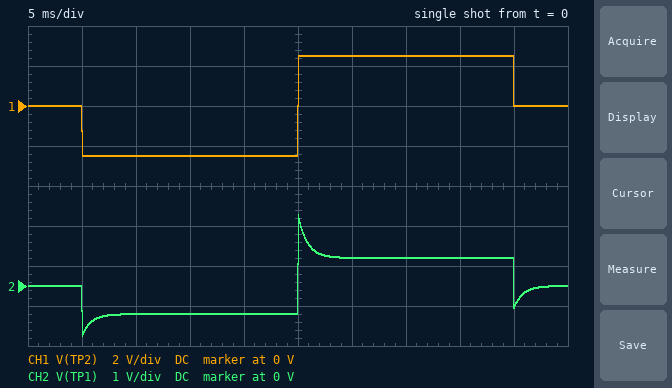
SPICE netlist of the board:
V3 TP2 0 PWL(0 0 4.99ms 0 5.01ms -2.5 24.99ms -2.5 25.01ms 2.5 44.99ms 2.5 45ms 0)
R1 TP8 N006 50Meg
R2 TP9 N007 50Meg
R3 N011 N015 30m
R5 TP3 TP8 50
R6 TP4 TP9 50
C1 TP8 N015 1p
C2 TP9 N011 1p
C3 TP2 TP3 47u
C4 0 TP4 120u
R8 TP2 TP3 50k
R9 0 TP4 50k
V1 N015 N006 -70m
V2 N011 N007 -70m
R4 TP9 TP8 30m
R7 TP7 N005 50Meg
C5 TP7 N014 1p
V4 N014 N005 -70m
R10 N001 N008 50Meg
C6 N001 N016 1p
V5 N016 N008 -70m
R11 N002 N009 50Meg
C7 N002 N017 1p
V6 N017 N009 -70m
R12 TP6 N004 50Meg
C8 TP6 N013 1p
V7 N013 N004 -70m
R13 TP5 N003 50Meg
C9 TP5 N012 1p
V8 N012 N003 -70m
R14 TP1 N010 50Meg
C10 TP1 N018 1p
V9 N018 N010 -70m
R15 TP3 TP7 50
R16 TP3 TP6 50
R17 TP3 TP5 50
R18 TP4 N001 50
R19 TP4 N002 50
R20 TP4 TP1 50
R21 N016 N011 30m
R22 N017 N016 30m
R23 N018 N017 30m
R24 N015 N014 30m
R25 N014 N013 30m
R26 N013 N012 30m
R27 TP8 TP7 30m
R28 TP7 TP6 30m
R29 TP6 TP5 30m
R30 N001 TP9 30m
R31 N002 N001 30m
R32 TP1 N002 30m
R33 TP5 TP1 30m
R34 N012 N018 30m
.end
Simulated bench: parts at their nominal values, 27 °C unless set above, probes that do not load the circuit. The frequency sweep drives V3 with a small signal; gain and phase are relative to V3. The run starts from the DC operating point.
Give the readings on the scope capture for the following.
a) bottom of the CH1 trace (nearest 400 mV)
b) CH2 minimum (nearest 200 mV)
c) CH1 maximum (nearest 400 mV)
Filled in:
-2.4 V
-1.2 V
2.4 V
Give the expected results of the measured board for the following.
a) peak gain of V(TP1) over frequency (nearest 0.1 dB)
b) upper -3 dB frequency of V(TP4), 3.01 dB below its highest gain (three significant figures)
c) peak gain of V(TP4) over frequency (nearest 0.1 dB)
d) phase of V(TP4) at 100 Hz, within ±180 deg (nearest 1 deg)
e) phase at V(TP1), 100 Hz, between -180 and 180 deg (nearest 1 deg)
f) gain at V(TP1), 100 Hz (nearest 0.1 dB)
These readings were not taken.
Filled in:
-6.0 dB
63.0 mHz
-6.0 dB
-28 deg
15 deg
-9.3 dB
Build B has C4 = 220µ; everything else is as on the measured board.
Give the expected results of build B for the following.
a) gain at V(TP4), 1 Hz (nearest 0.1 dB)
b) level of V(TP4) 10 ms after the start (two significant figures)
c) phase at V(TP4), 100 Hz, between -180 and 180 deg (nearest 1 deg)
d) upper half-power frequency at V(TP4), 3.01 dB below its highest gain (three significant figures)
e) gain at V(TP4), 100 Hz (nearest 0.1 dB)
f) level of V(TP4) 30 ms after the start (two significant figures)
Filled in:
-15.1 dB
-440 mV
-31 deg
27.5 mHz
-16.5 dB
430 mV
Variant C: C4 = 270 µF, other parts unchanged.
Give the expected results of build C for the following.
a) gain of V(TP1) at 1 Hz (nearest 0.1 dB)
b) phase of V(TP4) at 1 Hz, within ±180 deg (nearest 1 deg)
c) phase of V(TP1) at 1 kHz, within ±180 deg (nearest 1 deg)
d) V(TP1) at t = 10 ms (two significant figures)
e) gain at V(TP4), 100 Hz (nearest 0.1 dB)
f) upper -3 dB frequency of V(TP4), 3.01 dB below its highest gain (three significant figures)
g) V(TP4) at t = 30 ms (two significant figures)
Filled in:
-16.6 dB
-3 deg
6 deg
-380 mV
-18.0 dB
22.1 mHz
360 mV
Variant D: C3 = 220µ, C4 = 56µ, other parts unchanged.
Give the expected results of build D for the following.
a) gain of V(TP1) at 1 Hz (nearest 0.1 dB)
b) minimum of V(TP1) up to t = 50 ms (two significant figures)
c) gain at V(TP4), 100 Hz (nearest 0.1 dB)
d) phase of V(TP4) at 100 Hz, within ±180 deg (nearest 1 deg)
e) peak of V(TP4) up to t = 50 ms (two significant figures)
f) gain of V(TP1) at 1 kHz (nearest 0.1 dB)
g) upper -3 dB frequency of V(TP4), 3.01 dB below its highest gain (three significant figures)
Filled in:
-2.0 dB
-2.0 V
-3.7 dB
-35 deg
2.0 V
-5.9 dB
143 Hz
